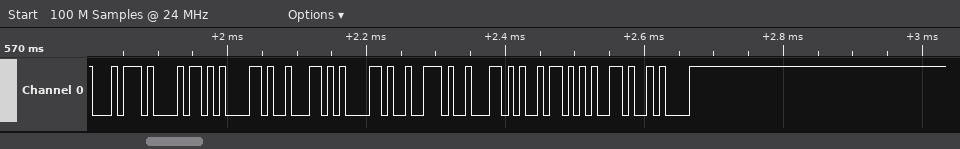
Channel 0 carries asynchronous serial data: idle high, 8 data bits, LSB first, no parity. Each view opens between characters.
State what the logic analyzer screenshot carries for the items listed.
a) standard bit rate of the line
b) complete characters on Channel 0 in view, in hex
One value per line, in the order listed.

115200 baud
74, 68, 61, 62, 61, 72, 62, 69, 65, 0A
